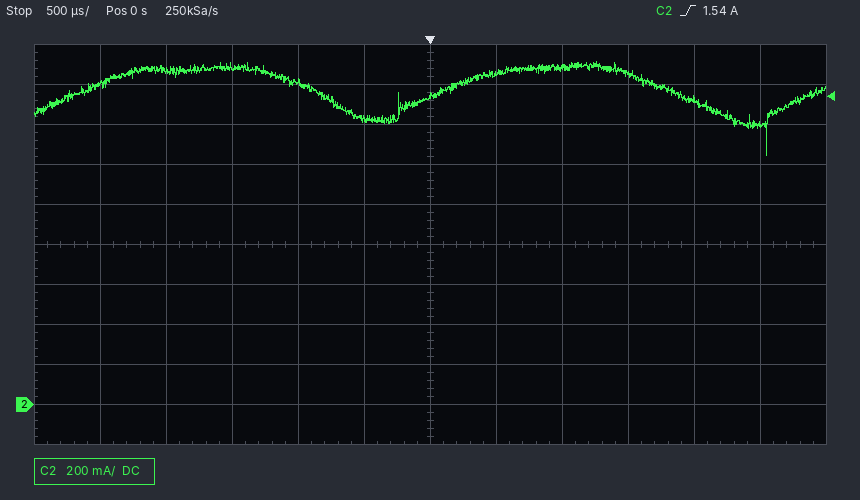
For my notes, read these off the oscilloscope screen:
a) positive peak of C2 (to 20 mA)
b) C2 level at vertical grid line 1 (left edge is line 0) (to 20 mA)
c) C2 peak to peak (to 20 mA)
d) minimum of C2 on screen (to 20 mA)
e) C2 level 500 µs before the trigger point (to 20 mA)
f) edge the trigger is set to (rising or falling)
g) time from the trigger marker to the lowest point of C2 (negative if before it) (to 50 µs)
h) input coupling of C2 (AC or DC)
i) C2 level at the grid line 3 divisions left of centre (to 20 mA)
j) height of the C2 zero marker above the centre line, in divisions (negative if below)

1.72 A
1.60 A
480 mA
1.24 A
1.42 A
rising
+2.55 ms
DC
1.68 A
-4.0 div
